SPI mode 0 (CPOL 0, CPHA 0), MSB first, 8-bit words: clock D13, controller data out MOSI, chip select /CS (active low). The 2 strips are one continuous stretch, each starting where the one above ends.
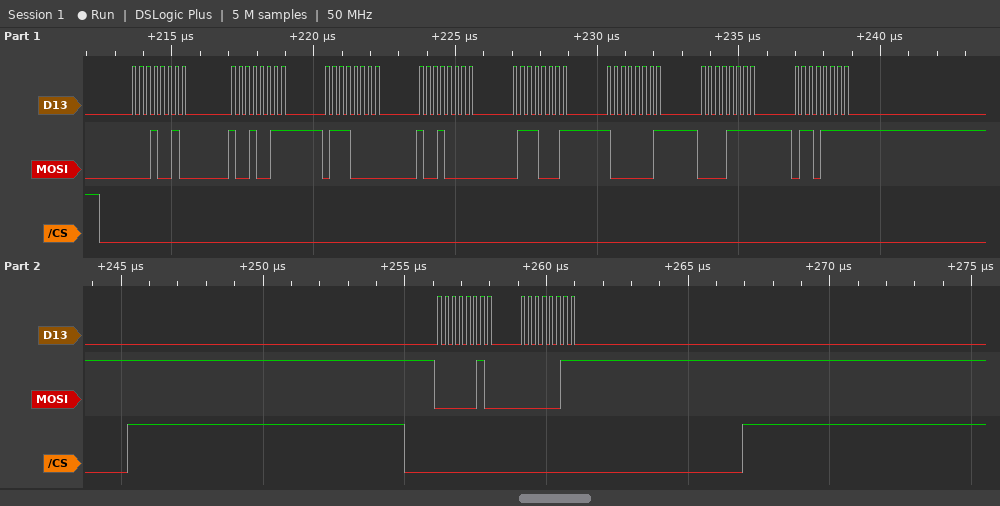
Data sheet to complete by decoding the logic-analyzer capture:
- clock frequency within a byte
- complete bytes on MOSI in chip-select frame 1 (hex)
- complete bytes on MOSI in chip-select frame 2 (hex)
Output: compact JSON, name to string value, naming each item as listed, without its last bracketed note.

{"clock frequency within a byte": "4 MHz", "complete bytes on MOSI in chip-select frame 1": "12 93 70 90 71 81 0F 6F", "complete bytes on MOSI in chip-select frame 2": "02 03"}
